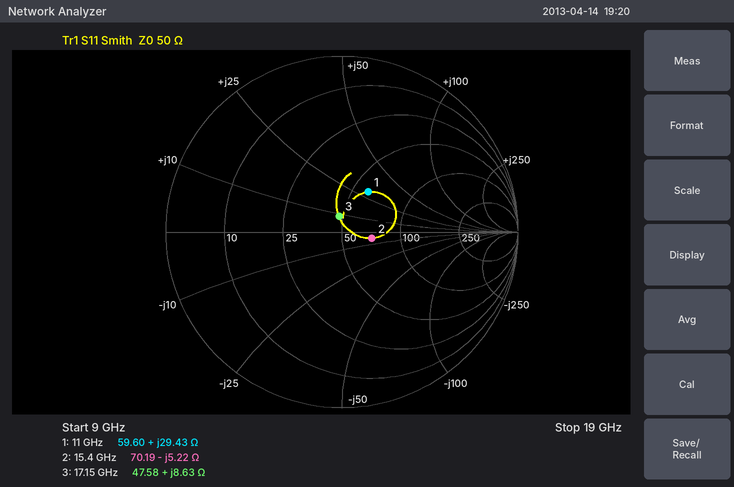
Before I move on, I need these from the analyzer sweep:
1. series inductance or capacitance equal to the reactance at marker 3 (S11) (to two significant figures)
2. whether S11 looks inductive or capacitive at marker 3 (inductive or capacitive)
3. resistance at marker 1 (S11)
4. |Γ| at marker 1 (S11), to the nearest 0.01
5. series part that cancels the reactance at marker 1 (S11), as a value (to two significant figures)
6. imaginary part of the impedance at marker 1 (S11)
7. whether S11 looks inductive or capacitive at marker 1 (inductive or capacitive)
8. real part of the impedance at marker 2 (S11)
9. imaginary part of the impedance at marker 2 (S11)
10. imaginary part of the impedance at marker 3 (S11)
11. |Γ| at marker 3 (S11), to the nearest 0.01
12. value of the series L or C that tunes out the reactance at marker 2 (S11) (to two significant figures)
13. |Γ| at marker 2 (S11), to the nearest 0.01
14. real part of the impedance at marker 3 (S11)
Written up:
80 pH
inductive
59.60 Ω
0.27
490 fF
+29.43 Ω
inductive
70.19 Ω
-5.22 Ω
+8.63 Ω
0.09
54 pH
0.17
47.58 Ω
